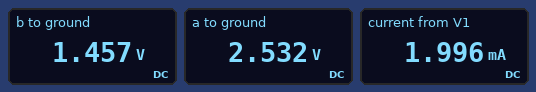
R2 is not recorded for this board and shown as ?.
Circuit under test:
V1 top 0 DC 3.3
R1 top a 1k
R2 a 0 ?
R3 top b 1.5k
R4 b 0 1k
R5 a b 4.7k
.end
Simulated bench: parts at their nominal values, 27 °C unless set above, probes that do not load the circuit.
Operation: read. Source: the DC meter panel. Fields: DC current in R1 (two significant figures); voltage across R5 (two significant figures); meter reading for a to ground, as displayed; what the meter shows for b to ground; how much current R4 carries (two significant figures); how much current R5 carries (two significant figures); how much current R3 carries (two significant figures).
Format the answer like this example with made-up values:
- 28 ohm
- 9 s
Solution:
- 770 µA
- 1.1 V
- 2.532 V
- 1.457 V
- 1.5 mA
- 230 µA
- 1.2 mA
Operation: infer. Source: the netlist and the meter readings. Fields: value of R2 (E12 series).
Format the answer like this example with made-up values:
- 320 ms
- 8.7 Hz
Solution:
- 4.7 kΩ
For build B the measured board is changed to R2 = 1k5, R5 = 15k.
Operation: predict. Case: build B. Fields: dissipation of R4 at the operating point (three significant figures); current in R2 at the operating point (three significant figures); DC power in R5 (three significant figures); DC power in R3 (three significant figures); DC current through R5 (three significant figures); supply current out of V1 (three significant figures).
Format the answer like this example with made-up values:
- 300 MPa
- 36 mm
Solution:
- 1.81 mW
- 1.30 mA
- 24.9 µW
- 2.55 mW
- 40.7 µA
- 2.65 mA
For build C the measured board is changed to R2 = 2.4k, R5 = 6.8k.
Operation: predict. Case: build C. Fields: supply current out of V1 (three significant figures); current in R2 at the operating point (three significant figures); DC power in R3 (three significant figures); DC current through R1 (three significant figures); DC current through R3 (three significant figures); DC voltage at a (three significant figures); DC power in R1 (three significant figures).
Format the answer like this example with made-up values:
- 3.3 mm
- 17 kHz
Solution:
- 2.33 mA
- 934 µA
- 2.42 mW
- 1.06 mA
- 1.27 mA
- 2.24 V
- 1.12 mW
